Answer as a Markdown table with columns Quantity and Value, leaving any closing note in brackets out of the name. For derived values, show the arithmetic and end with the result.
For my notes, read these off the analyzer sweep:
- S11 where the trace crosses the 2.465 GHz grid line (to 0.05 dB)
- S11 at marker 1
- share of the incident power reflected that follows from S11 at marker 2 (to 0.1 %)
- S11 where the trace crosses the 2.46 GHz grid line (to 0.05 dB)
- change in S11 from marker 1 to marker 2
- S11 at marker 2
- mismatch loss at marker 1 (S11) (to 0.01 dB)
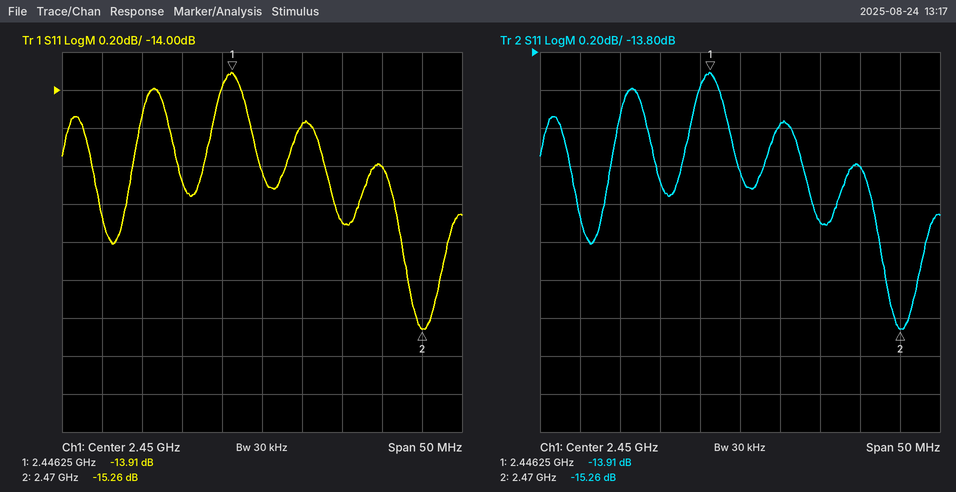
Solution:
| Quantity | Value |
|---|---|
| S11 where the trace crosses the 2.465 GHz grid line | -14.40 dB |
| S11 at marker 1 | -13.91 dB |
| share of the incident power reflected that follows from S11 at marker 2 | 10^(-15.26/10) ≈ 3.0 % |
| S11 where the trace crosses the 2.46 GHz grid line | -14.70 dB |
| change in S11 from marker 1 to marker 2 | -15.26 − (-13.91) = -1.35 dB |
| S11 at marker 2 | -15.26 dB |
| mismatch loss at marker 1 (S11) | −10 log10(1 − 10^(-13.91/10)) ≈ 0.18 dB |
